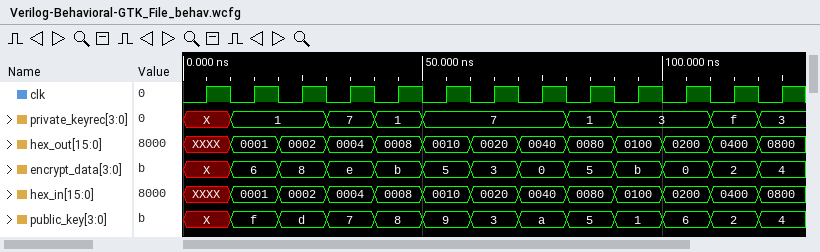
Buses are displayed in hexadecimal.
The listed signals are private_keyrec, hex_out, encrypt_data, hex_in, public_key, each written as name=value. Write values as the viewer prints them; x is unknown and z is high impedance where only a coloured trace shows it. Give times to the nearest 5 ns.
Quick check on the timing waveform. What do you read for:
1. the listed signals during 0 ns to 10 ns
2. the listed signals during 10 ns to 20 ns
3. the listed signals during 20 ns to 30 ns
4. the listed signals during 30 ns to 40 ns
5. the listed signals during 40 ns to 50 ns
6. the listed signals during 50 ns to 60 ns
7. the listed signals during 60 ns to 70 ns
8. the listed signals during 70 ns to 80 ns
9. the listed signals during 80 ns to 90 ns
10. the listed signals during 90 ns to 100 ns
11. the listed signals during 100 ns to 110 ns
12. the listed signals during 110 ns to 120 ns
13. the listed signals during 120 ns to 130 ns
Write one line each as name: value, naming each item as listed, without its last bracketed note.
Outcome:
the listed signals during 0 ns to 10 ns: private_keyrec=X, hex_out=XXXX, encrypt_data=X, hex_in=XXXX, public_key=X
the listed signals during 10 ns to 20 ns: private_keyrec=1, hex_out=0001, encrypt_data=6, hex_in=0001, public_key=f
the listed signals during 20 ns to 30 ns: private_keyrec=1, hex_out=0002, encrypt_data=8, hex_in=0002, public_key=d
the listed signals during 30 ns to 40 ns: private_keyrec=7, hex_out=0004, encrypt_data=e, hex_in=0004, public_key=7
the listed signals during 40 ns to 50 ns: private_keyrec=1, hex_out=0008, encrypt_data=b, hex_in=0008, public_key=8
the listed signals during 50 ns to 60 ns: private_keyrec=7, hex_out=0010, encrypt_data=5, hex_in=0010, public_key=9
the listed signals during 60 ns to 70 ns: private_keyrec=7, hex_out=0020, encrypt_data=3, hex_in=0020, public_key=3
the listed signals during 70 ns to 80 ns: private_keyrec=7, hex_out=0040, encrypt_data=0, hex_in=0040, public_key=a
the listed signals during 80 ns to 90 ns: private_keyrec=1, hex_out=0080, encrypt_data=5, hex_in=0080, public_key=5
the listed signals during 90 ns to 100 ns: private_keyrec=3, hex_out=0100, encrypt_data=b, hex_in=0100, public_key=1
the listed signals during 100 ns to 110 ns: private_keyrec=3, hex_out=0200, encrypt_data=0, hex_in=0200, public_key=6
the listed signals during 110 ns to 120 ns: private_keyrec=f, hex_out=0400, encrypt_data=2, hex_in=0400, public_key=2
the listed signals during 120 ns to 130 ns: private_keyrec=3, hex_out=0800, encrypt_data=4, hex_in=0800, public_key=4
